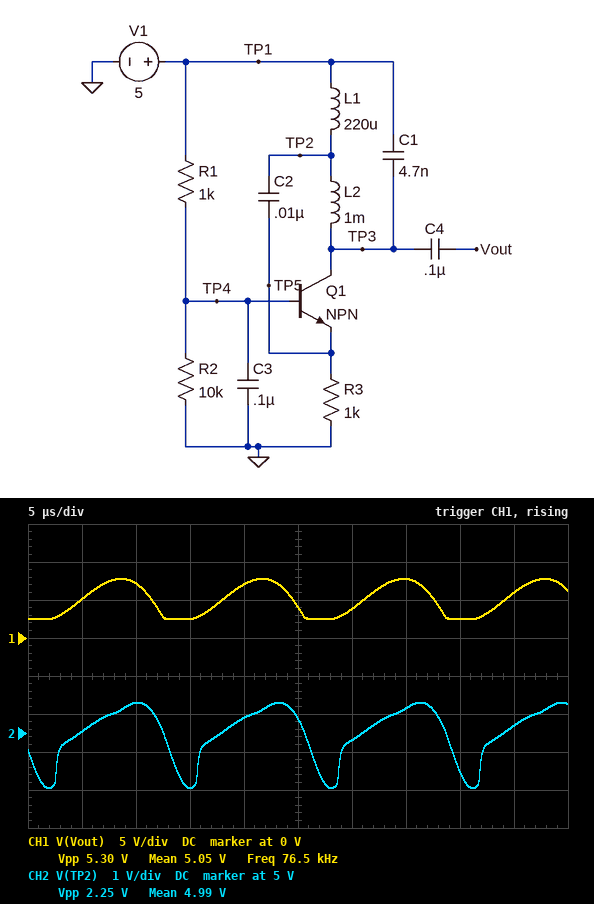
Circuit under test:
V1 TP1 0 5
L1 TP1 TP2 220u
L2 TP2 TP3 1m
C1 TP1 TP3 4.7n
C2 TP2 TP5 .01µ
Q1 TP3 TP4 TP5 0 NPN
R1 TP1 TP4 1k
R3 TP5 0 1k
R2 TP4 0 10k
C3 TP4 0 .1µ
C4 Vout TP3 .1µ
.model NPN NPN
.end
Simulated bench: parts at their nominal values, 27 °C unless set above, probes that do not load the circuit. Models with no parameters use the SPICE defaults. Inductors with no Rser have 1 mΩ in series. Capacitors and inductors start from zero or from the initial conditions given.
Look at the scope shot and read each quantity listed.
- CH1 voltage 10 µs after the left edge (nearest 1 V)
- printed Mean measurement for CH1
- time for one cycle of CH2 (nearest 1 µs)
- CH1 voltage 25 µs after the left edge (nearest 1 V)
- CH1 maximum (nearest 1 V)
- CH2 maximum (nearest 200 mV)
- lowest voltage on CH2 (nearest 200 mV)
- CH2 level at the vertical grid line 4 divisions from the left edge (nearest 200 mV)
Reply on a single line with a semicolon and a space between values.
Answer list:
7 V; 5.05 V; 13 µs; 4 V; 8 V; 5.8 V; 3.6 V; 5.4 V
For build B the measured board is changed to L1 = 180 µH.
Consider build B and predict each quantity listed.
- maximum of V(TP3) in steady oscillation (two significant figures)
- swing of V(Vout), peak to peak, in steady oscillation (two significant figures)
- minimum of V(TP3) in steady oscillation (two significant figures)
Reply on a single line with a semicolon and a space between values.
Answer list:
6.9 V; 3.7 V; 3.2 V
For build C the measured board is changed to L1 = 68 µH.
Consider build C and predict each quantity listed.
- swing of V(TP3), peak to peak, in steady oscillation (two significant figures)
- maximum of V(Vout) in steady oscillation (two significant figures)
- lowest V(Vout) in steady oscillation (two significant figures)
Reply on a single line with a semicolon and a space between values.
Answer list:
2.4 V; 6.2 V; 3.8 V
